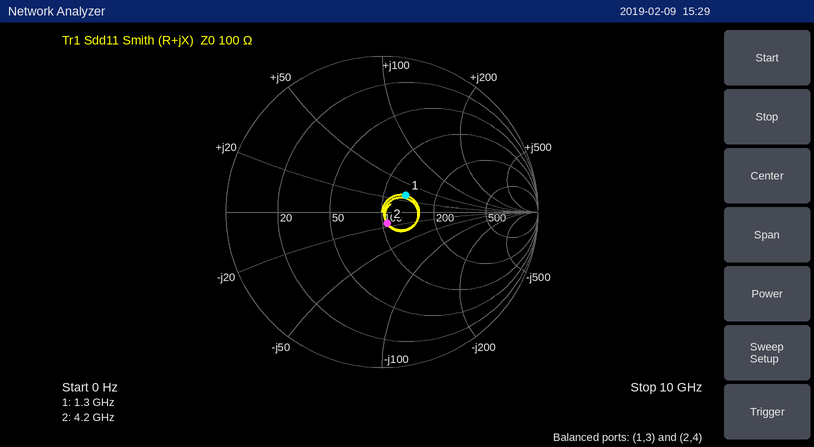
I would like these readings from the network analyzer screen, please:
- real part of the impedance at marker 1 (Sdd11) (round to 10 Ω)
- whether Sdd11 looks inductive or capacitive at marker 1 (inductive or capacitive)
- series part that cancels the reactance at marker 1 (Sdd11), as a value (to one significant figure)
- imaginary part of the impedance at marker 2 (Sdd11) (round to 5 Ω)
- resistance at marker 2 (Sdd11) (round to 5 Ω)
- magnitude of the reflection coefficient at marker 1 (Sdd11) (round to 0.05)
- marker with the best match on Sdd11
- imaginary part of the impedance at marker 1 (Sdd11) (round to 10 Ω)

130 Ω
inductive
4 pF
-15 Ω
105 Ω
0.20
marker 2
+30 Ω
